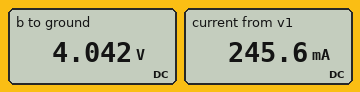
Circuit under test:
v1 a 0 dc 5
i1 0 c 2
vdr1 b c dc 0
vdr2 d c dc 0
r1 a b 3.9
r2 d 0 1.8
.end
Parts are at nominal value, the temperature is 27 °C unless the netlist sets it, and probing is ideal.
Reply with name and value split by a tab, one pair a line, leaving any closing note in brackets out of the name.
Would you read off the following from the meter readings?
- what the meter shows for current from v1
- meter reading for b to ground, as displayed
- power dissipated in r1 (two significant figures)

what the meter shows for current from v1	245.6 mA
meter reading for b to ground, as displayed	4.042 V
power dissipated in r1	240 mW
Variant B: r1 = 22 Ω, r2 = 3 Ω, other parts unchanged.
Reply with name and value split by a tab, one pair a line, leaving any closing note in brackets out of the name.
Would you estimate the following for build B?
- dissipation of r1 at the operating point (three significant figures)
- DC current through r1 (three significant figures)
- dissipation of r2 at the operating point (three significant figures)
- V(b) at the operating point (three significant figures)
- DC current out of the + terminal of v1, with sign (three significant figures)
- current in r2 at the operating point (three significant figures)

dissipation of r1 at the operating point	35.2 mW
DC current through r1	40.0 mA
dissipation of r2 at the operating point	11.5 W
V(b) at the operating point	5.88 V
DC current out of the + terminal of v1, with sign	-40.0 mA
current in r2 at the operating point	1.96 A
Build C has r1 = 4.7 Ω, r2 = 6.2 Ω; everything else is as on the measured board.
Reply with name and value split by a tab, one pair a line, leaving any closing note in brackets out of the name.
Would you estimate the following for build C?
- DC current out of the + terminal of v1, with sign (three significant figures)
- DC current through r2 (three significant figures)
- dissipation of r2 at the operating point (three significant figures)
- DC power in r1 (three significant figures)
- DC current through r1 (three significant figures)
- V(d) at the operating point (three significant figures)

DC current out of the + terminal of v1, with sign	-679 mA
DC current through r2	1.32 A
dissipation of r2 at the operating point	10.8 W
DC power in r1	2.17 W
DC current through r1	679 mA
V(d) at the operating point	8.19 V
